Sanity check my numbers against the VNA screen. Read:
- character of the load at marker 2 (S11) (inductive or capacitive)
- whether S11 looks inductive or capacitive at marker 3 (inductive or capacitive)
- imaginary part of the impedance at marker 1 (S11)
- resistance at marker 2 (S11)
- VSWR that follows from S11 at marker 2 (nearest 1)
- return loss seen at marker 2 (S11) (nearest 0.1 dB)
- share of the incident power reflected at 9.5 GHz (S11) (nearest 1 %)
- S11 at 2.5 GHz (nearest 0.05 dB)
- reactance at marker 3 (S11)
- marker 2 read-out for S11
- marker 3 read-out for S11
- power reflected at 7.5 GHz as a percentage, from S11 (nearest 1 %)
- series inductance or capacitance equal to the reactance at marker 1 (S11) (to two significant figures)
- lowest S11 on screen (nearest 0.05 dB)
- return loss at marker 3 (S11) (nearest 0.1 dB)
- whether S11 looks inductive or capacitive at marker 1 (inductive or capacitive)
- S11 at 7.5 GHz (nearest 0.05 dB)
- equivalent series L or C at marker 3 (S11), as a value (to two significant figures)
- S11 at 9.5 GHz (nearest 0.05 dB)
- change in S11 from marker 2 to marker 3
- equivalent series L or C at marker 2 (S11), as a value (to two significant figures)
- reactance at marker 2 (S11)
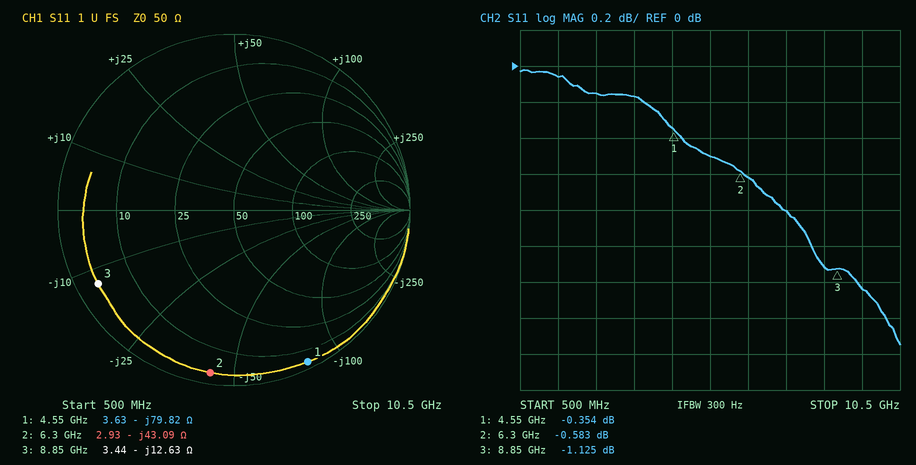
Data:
capacitive
capacitive
-79.82 Ω
2.93 Ω
30
0.6 dB
75 %
-0.15 dB
-12.63 Ω
-0.583 dB
-1.125 dB
83 %
440 fF
-1.55 dB
1.1 dB
capacitive
-0.80 dB
1.4 pF
-1.25 dB
-0.542 dB
590 fF
-43.09 Ω
